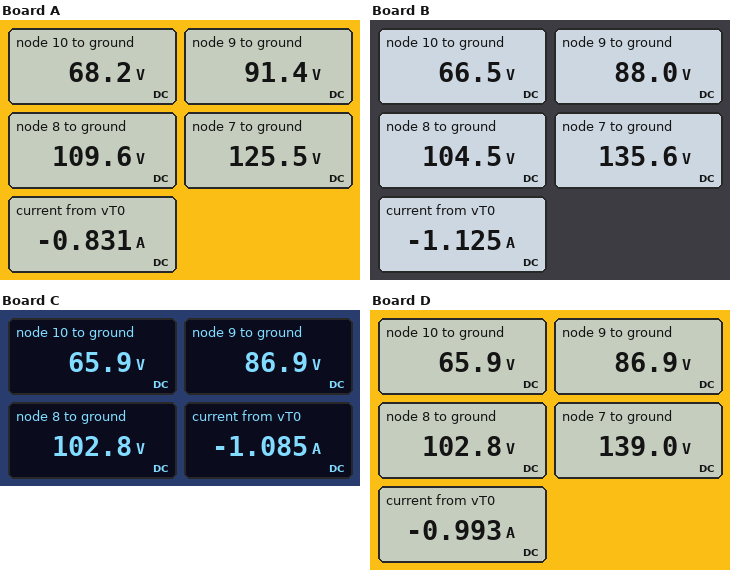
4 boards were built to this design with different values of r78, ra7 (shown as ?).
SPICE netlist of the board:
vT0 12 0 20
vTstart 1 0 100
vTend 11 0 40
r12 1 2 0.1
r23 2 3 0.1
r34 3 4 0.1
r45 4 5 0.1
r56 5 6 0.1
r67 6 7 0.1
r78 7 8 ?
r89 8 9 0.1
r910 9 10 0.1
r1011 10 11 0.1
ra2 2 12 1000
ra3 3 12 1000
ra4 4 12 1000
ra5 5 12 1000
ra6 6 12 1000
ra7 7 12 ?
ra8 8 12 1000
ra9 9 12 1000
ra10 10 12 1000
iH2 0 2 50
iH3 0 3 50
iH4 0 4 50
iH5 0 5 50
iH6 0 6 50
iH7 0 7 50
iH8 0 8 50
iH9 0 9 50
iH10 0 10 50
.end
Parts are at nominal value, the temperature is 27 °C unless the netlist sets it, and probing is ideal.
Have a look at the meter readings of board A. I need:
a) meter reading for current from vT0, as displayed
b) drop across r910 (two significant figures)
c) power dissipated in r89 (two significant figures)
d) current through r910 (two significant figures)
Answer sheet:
-0.831 A
23 V
3.3 kW
230 A
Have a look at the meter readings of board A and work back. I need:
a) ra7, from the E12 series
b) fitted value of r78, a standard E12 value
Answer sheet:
1.5 kΩ
0.12 Ω
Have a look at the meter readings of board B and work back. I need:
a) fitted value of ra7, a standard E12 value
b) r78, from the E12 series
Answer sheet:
330 Ω
0.27 Ω
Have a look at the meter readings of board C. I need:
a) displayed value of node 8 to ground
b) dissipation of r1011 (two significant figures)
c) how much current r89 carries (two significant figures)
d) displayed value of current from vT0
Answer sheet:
102.8 V
6.7 kW
160 A
-1.085 A
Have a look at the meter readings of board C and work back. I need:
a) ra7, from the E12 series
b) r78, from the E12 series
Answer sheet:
390 Ω
0.33 Ω
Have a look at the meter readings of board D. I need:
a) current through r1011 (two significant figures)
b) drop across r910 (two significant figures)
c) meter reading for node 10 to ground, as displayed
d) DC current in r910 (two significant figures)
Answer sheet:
260 A
21 V
65.9 V
210 A
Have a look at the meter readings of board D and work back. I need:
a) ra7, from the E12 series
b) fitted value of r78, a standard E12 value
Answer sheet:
560 Ω
0.33 Ω
